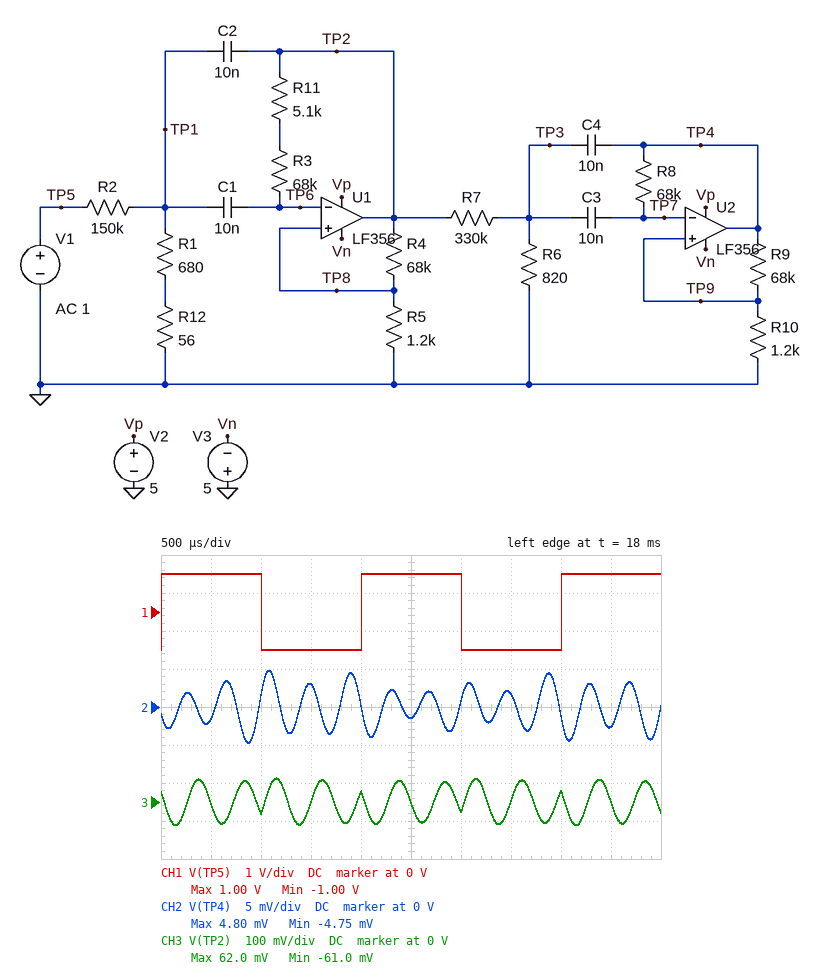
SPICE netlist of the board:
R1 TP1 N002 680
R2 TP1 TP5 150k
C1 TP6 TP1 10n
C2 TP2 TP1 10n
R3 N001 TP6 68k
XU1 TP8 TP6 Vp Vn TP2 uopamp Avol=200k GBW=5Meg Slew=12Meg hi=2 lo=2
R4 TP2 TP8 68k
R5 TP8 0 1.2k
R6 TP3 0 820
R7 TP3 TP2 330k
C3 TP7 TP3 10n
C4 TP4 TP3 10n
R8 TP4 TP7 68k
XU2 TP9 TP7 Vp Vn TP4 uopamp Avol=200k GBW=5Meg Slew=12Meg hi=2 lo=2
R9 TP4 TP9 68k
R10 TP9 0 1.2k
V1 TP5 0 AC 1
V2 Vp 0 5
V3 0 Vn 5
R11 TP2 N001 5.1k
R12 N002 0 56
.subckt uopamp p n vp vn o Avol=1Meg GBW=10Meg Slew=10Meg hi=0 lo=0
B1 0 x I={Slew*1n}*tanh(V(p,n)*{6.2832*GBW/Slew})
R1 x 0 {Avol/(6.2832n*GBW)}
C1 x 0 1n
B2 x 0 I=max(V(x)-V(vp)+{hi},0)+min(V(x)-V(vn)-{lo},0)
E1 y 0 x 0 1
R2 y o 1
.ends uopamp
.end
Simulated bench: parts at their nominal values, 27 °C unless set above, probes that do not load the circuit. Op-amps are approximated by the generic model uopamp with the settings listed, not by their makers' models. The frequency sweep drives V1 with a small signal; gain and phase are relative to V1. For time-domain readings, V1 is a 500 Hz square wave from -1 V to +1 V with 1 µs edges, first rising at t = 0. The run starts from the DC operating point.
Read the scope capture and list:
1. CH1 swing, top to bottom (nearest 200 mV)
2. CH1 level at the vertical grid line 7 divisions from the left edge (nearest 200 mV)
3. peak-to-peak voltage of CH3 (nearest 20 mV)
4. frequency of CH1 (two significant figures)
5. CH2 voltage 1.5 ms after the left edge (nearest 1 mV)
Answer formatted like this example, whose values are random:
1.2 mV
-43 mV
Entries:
2.0 V
-1.0 V
120 mV
500 Hz
3 mV
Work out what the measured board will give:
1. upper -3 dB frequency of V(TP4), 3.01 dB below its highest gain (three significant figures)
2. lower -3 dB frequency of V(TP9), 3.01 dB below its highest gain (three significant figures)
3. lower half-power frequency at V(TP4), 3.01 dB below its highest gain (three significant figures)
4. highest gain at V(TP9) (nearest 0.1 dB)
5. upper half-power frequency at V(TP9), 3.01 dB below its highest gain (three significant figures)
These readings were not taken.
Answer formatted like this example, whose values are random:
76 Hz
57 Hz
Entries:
2.19 kHz
2.14 kHz
2.14 kHz
-38.4 dB
2.19 kHz
